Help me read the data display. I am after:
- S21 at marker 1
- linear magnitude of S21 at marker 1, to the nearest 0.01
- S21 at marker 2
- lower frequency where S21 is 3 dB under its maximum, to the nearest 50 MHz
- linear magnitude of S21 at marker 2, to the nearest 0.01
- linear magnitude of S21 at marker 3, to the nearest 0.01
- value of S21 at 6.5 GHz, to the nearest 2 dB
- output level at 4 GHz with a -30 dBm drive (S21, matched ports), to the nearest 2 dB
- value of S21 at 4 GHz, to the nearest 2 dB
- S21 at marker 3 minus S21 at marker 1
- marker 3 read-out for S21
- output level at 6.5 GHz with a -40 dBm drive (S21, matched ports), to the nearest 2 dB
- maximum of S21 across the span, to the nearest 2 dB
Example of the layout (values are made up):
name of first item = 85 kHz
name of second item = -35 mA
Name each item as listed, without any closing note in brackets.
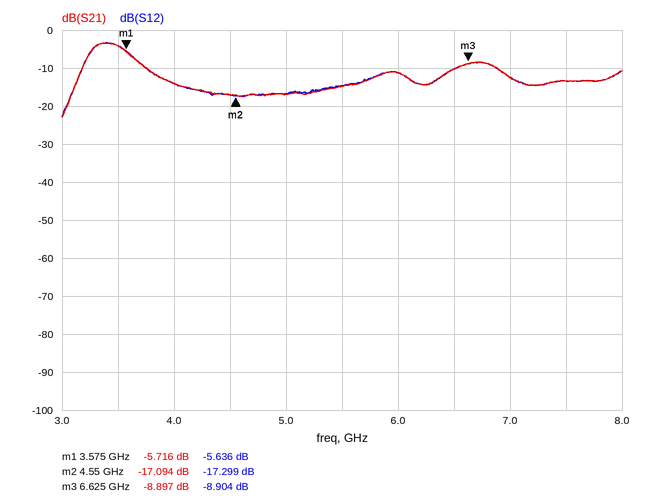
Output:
S21 at marker 1 = -5.716 dB
linear magnitude of S21 at marker 1, to the nearest 0.01 = 0.52
S21 at marker 2 = -17.094 dB
lower frequency where S21 is 3 dB under its maximum, to the nearest 50 MHz = 3.25 GHz
linear magnitude of S21 at marker 2, to the nearest 0.01 = 0.14
linear magnitude of S21 at marker 3, to the nearest 0.01 = 0.36
value of S21 at 6.5 GHz, to the nearest 2 dB = -10 dB
output level at 4 GHz with a -30 dBm drive (S21, matched ports), to the nearest 2 dB = -44 dBm
value of S21 at 4 GHz, to the nearest 2 dB = -14 dB
S21 at marker 3 minus S21 at marker 1 = -3.181 dB
marker 3 read-out for S21 = -8.897 dB
output level at 6.5 GHz with a -40 dBm drive (S21, matched ports), to the nearest 2 dB = -50 dBm
maximum of S21 across the span, to the nearest 2 dB = -4 dB
